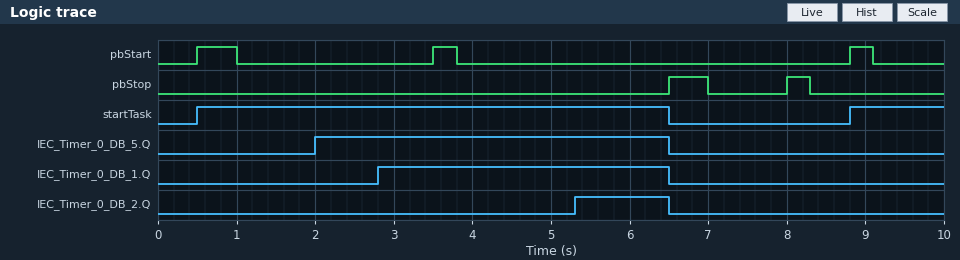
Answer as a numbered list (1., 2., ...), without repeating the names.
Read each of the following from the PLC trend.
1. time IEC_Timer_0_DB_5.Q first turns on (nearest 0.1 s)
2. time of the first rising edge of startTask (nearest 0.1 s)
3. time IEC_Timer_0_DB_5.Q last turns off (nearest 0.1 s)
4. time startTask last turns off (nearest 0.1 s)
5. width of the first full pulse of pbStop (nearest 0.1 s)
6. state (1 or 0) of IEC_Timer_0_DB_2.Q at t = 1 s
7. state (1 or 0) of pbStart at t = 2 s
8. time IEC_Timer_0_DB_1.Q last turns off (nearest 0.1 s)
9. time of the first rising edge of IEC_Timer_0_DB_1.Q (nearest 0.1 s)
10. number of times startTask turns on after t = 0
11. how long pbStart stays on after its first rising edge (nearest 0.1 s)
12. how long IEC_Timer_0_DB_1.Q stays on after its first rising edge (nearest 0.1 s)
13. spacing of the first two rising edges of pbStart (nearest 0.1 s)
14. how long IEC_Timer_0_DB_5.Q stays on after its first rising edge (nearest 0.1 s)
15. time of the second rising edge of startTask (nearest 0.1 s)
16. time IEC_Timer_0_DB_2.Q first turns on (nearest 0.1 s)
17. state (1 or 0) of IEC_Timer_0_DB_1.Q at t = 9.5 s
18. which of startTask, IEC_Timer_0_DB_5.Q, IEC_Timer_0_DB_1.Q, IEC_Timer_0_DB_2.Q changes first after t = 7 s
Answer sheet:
1. 2.0 s
2. 0.5 s
3. 6.5 s
4. 6.5 s
5. 0.5 s
6. 0
7. 0
8. 6.5 s
9. 2.8 s
10. 2
11. 0.5 s
12. 3.7 s
13. 3.0 s
14. 4.5 s
15. 8.8 s
16. 5.3 s
17. 0
18. startTask
